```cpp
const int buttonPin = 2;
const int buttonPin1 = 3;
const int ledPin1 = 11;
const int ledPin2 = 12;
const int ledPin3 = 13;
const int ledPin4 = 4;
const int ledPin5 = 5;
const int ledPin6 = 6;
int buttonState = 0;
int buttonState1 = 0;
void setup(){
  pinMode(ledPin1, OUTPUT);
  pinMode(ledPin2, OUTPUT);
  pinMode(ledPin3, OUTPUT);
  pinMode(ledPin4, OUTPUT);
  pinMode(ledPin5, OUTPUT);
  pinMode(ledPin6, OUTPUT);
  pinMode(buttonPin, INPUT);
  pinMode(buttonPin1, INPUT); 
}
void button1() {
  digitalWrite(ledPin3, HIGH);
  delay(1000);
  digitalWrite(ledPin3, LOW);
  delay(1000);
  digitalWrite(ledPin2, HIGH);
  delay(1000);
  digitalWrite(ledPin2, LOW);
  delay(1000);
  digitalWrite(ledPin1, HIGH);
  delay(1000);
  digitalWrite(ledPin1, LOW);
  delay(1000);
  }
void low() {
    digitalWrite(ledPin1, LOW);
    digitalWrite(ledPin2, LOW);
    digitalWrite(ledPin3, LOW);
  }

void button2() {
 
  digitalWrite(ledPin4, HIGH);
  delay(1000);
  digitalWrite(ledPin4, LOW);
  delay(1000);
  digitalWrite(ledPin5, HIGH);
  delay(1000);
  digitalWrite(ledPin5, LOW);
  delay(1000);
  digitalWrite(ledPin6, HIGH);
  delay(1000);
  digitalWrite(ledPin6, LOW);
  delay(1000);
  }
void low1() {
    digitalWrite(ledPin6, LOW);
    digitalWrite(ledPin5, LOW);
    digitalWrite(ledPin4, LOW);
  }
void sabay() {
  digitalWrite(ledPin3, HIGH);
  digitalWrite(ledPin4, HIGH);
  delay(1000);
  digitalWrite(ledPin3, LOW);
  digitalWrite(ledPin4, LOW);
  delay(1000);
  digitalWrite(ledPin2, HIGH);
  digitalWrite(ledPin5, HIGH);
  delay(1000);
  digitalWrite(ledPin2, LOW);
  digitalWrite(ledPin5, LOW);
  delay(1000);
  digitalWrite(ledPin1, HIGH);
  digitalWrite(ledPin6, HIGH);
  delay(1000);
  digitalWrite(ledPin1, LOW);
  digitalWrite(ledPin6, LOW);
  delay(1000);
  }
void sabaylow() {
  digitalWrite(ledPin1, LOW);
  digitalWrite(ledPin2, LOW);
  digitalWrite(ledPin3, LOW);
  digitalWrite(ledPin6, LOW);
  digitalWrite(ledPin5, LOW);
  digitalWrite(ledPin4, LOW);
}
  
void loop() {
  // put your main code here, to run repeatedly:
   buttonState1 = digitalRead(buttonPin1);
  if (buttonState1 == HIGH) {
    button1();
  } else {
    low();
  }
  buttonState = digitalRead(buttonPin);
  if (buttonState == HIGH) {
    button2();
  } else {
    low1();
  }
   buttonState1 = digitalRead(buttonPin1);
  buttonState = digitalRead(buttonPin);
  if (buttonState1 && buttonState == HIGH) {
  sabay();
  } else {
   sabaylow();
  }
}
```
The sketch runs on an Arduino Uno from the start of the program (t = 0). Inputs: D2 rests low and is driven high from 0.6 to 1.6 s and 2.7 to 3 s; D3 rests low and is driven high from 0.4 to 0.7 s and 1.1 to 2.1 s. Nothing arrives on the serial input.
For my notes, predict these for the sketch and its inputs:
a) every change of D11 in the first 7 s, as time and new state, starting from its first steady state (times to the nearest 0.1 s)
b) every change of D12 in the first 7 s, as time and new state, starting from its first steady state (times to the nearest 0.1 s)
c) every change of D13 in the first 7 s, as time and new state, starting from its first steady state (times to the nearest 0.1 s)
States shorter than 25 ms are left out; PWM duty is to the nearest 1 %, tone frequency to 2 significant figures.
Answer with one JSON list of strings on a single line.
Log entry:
["0 s low; 4.4 s high; 5.4 s low", "0 s low; 2.4 s high; 3.4 s low", "0 s low; 0.4 s high; 1.4 s low"]
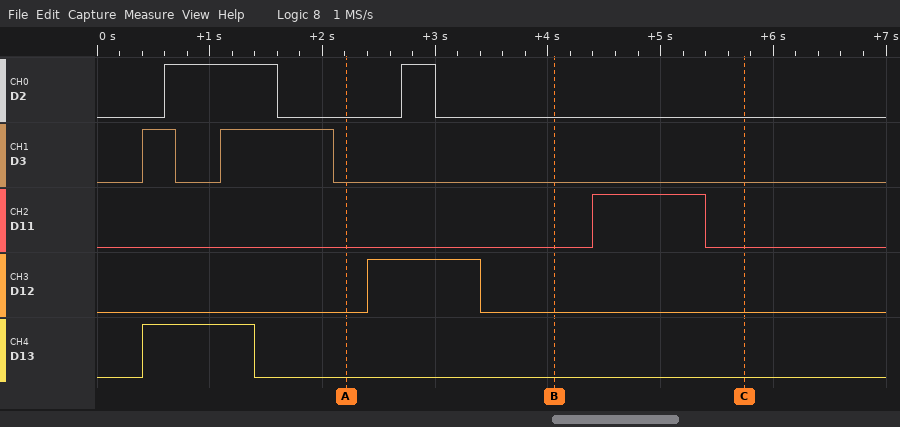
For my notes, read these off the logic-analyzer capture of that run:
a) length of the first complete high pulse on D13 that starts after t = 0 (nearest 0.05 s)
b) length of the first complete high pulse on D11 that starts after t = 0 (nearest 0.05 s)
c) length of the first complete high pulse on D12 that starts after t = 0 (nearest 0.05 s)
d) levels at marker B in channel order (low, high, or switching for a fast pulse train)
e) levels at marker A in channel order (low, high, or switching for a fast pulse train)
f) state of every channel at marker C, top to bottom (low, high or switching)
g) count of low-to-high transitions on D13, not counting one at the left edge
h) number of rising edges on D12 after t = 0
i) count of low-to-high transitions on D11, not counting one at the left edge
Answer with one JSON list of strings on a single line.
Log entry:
["1.00 s", "1.00 s", "1.00 s", "D2 low, D3 low, D11 low, D12 low, D13 low", "D2 low, D3 low, D11 low, D12 low, D13 low", "D2 low, D3 low, D11 low, D12 low, D13 low", "1", "1", "1"]
